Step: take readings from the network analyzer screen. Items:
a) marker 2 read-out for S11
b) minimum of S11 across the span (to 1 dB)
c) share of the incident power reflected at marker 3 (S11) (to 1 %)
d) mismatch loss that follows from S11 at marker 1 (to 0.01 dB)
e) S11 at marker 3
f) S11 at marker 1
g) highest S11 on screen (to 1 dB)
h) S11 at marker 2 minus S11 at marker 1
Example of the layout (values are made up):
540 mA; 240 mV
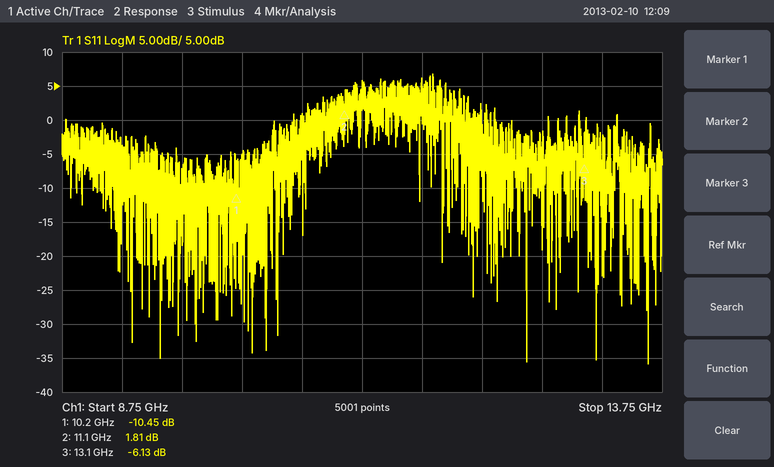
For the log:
1.81 dB; -36 dB; 24 %; 0.41 dB; -6.13 dB; -10.45 dB; 7 dB; 12.26 dB
